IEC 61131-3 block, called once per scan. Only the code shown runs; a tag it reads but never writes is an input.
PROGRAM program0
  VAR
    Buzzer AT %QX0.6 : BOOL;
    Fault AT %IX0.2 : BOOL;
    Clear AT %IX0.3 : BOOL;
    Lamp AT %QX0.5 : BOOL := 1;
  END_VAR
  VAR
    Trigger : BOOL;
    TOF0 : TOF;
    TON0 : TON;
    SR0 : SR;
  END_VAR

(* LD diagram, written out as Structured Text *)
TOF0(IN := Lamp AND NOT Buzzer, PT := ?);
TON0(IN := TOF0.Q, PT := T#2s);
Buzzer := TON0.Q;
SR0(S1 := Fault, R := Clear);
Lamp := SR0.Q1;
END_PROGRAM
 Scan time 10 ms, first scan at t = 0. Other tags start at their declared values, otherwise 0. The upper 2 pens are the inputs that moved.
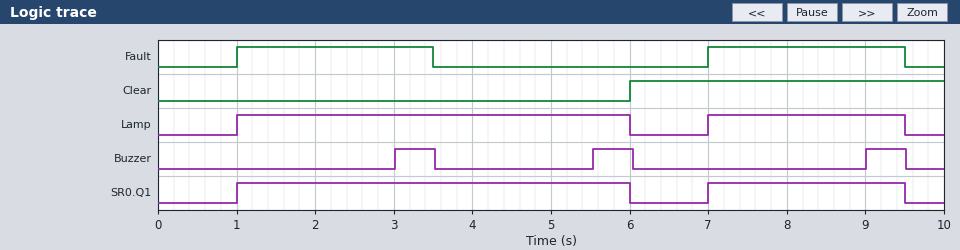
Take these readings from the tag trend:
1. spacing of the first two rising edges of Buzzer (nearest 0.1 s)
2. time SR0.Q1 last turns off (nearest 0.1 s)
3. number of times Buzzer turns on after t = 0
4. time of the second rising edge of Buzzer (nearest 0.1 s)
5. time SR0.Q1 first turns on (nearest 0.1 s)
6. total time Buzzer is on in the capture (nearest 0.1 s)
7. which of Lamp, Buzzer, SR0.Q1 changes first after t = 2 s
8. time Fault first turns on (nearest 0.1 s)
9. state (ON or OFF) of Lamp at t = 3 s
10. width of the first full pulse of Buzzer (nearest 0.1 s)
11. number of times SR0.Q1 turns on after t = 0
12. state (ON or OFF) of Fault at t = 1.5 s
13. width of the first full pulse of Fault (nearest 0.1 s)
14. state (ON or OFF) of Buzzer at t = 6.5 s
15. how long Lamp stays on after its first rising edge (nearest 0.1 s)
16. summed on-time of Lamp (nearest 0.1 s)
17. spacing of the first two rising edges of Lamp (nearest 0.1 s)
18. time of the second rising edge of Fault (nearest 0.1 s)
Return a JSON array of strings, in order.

["2.5 s", "9.5 s", "3", "5.5 s", "1.0 s", "1.5 s", "Buzzer", "1.0 s", "ON", "0.5 s", "2", "ON", "2.5 s", "OFF", "5.0 s", "7.5 s", "6.0 s", "7.0 s"]
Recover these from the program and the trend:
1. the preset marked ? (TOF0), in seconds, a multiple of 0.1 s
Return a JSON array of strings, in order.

["0.5 s"]
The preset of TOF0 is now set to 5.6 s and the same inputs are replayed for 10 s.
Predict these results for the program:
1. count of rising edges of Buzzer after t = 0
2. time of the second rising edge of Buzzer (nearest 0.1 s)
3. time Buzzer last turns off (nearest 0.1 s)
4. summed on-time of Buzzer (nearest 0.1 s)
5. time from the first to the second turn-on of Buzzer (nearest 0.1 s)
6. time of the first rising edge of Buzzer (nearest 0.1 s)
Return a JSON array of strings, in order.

["2", "9.6 s", "7.6 s", "6.0 s", "7.6 s", "2.0 s"]
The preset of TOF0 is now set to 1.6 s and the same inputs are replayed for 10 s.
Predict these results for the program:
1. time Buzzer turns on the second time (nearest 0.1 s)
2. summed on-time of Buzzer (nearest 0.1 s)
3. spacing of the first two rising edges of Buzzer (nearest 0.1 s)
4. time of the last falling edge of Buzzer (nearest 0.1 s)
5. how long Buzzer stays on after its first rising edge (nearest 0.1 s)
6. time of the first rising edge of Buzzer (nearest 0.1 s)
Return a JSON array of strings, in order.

["5.6 s", "4.0 s", "3.6 s", "7.2 s", "1.6 s", "2.0 s"]
